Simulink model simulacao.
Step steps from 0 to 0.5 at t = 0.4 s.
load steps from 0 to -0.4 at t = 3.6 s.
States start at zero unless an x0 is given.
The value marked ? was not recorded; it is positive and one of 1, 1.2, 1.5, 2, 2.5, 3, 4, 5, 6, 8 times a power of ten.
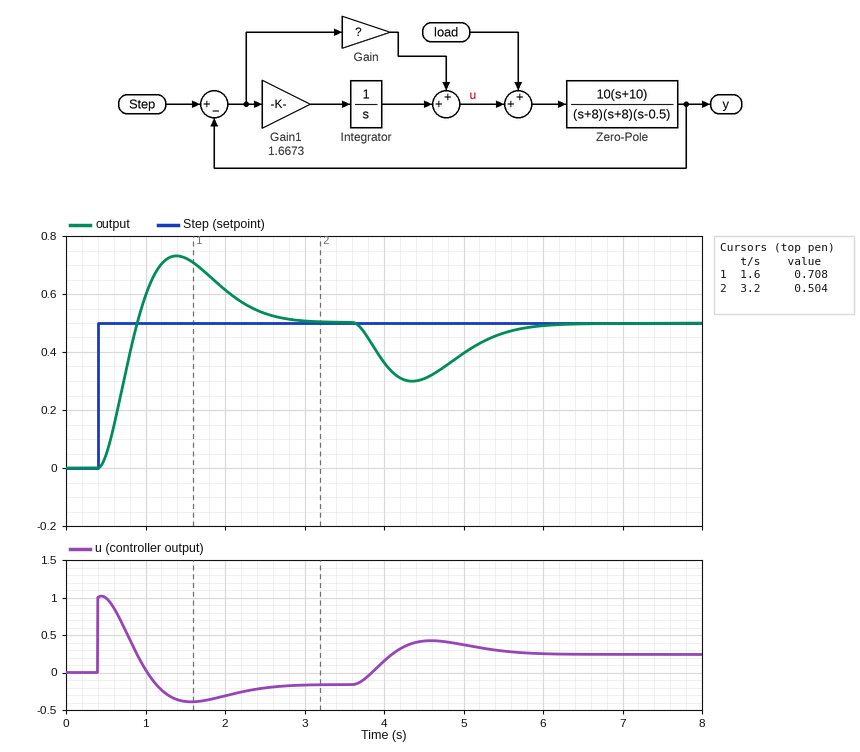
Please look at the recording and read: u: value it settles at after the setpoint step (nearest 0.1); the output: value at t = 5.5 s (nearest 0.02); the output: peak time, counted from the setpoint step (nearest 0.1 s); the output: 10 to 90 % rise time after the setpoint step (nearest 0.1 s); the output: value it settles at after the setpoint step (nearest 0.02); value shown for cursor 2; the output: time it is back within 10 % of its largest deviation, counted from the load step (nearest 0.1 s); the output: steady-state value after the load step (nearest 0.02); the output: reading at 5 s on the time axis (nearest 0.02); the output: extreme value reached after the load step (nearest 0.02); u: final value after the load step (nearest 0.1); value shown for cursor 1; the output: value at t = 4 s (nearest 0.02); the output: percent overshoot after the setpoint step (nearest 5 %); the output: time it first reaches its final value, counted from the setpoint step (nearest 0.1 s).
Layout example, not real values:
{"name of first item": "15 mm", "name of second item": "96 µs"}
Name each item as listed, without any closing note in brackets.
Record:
{"u: value it settles at after the setpoint step": "-0.2", "the output: value at t = 5.5 s": "0.46", "the output: peak time, counted from the setpoint step": "1.0 s", "the output: 10 to 90 % rise time after the setpoint step": "0.3 s", "the output: value it settles at after the setpoint step": "0.50", "value shown for cursor 2": "0.504", "the output: time it is back within 10 % of its largest deviation, counted from the load step": "2.1 s", "the output: steady-state value after the load step": "0.50", "the output: reading at 5 s on the time axis": "0.40", "the output: extreme value reached after the load step": "0.30", "u: final value after the load step": "0.2", "value shown for cursor 1": "0.708", "the output: value at t = 4 s": "0.36", "the output: percent overshoot after the setpoint step": "45 %", "the output: time it first reaches its final value, counted from the setpoint step": "0.5 s"}
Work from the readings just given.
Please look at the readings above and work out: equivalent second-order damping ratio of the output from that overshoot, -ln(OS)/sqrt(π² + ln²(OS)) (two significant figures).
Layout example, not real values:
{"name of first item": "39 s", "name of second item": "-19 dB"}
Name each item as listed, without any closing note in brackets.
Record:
{"equivalent second-order damping ratio of the output from that overshoot, -ln(OS)/sqrt(π² + ln²(OS))": "0.25"}
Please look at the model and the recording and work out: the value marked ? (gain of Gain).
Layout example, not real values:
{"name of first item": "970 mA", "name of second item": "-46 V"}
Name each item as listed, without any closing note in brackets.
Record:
{"the value marked ?": "2"}
